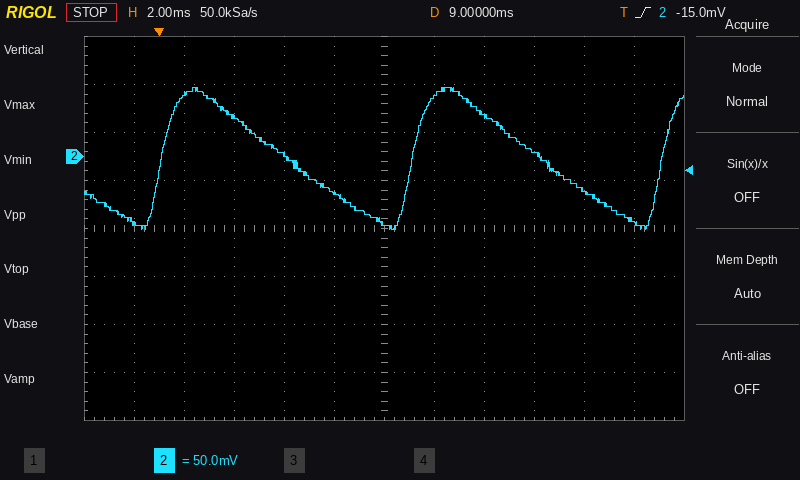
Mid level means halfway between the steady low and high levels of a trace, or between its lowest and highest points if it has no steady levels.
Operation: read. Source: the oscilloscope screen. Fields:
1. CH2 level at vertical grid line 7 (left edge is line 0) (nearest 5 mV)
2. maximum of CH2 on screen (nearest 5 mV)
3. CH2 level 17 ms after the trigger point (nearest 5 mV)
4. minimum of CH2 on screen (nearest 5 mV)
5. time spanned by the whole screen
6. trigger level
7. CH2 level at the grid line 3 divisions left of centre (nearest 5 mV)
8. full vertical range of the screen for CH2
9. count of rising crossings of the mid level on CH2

65 mV
70 mV
-35 mV
-75 mV
24 ms
-15.0 mV
40 mV
400 mV
3
